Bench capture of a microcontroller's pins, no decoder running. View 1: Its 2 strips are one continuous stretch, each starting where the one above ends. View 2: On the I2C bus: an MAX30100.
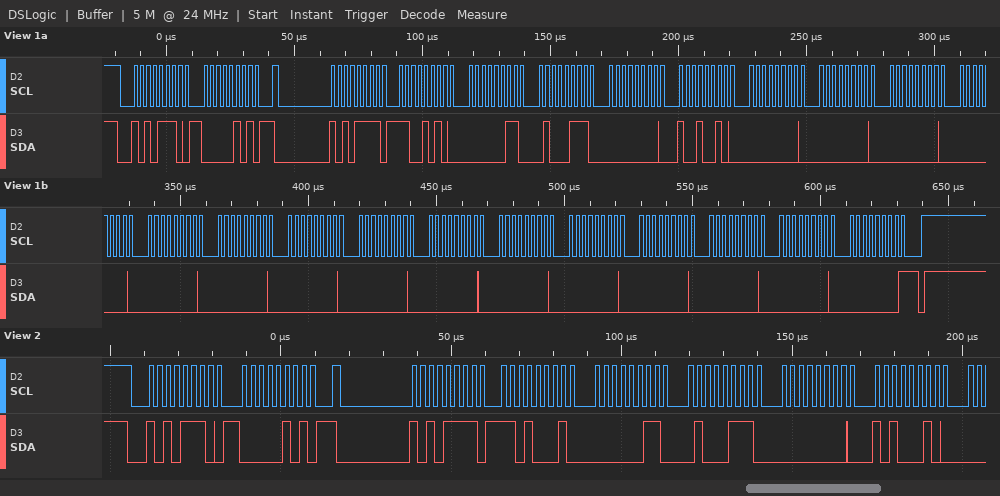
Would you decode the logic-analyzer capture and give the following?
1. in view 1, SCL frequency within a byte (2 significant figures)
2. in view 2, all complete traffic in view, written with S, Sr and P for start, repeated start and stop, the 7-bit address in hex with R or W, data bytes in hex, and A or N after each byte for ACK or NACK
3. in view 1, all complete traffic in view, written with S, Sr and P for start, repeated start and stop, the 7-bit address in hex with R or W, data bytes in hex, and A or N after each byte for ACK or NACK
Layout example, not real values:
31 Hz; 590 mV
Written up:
400 kHz; S 57W A 05 A Sr 57R A D1 A 03 A 47 A 00 A A2 A; S 57W A 05 A Sr 57R A CA A 03 A 47 A 00 A 92 A 00 A 00 A 00 A 00 A 00 A 00 A 00 A 00 A 00 A 00 A 00 A 00 A 00 A 00 A 00 N P
